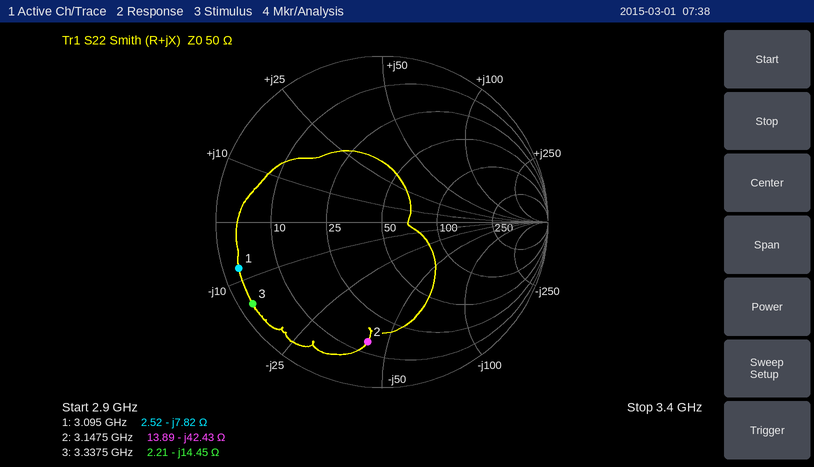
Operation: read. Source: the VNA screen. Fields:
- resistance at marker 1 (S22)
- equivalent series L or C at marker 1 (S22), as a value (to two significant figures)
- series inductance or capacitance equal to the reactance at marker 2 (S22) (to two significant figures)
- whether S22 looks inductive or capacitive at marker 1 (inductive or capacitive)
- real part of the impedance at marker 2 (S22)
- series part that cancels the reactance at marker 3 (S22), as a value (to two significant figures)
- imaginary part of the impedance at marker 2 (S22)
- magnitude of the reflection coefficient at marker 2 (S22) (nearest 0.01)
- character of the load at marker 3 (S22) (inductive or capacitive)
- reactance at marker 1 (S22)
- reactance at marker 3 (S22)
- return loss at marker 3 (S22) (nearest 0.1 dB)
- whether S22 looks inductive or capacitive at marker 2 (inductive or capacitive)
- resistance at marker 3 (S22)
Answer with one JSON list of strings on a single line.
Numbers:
["2.52 Ω", "6.6 pF", "1.2 pF", "capacitive", "13.89 Ω", "690 pH", "-42.43 Ω", "0.73", "capacitive", "-7.82 Ω", "-14.45 Ω", "0.7 dB", "capacitive", "2.21 Ω"]
